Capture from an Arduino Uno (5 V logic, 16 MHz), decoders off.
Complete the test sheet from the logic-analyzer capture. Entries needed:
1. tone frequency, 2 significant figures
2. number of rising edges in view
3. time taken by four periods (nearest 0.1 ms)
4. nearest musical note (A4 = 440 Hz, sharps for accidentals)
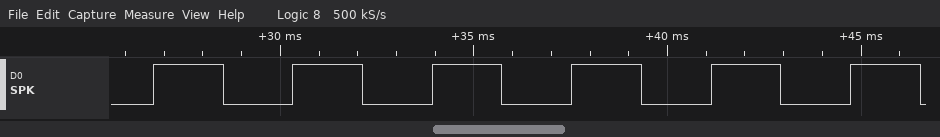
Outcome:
280 Hz
6
14.4 ms
C#4
